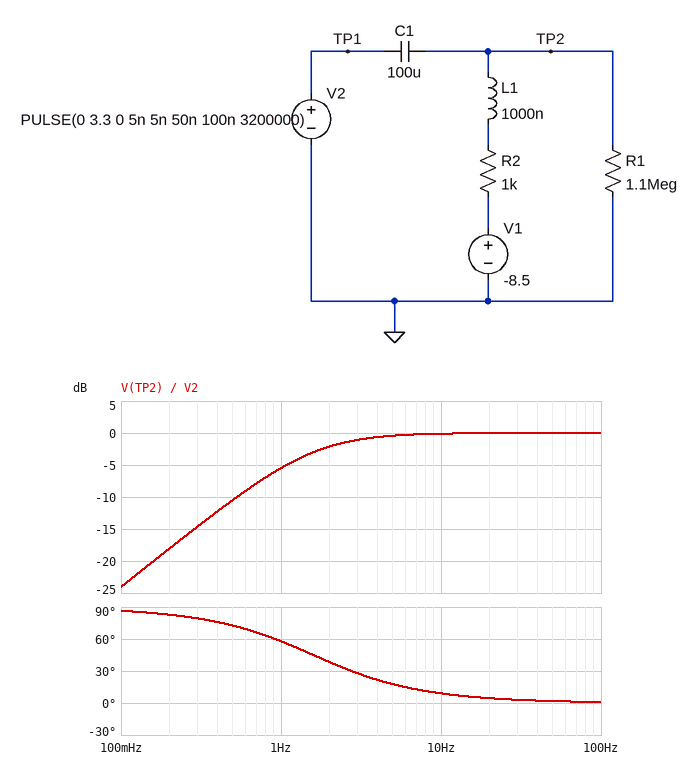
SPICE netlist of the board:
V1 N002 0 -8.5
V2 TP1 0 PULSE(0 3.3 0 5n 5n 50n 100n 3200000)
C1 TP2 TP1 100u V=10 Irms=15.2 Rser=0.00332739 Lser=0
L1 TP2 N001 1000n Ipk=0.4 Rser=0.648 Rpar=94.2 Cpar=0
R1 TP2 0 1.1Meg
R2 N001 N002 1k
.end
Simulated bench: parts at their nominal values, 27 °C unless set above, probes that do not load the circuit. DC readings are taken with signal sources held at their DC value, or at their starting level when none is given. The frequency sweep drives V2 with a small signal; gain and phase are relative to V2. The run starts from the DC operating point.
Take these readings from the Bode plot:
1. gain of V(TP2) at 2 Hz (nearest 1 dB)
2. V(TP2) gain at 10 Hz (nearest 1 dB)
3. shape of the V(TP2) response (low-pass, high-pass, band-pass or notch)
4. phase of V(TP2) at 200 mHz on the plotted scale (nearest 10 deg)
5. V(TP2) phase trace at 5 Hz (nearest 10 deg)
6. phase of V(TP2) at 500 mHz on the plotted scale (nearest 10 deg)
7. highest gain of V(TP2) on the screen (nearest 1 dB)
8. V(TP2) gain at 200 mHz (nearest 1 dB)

-2 dB
0 dB
high-pass
80 deg
20 deg
70 deg
0 dB
-18 dB
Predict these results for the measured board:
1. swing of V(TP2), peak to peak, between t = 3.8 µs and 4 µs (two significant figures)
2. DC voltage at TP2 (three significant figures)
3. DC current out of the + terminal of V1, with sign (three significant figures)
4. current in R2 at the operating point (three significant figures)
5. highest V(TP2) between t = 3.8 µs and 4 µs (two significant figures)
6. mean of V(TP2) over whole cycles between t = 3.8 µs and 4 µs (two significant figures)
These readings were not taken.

3.3 V
-8.49 V
-7.72 µA
7.72 µA
-5.2 V
-6.7 V
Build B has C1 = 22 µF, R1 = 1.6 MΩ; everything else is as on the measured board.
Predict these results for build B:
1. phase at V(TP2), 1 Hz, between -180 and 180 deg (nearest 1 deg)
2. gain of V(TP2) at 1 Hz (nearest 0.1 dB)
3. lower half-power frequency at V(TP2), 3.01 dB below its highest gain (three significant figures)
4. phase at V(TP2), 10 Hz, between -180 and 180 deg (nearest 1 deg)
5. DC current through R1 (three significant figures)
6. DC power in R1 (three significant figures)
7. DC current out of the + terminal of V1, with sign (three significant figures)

82 deg
-17.3 dB
7.23 Hz
36 deg
5.31 µA
45.1 µW
-5.31 µA
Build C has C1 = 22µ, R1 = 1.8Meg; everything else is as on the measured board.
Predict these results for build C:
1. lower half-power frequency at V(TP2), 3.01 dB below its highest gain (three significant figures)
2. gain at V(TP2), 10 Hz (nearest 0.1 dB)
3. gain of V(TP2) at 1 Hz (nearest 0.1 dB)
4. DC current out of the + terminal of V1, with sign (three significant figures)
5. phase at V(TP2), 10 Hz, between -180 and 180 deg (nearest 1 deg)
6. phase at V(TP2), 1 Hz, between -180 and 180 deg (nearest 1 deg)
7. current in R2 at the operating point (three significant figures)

7.23 Hz
-1.8 dB
-17.3 dB
-4.72 µA
36 deg
82 deg
4.72 µA
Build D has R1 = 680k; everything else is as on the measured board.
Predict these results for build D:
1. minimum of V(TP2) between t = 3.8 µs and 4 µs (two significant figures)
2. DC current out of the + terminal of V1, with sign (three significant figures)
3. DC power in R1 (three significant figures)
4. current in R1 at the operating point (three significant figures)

-8.5 V
-12.5 µA
106 µW
12.5 µA
